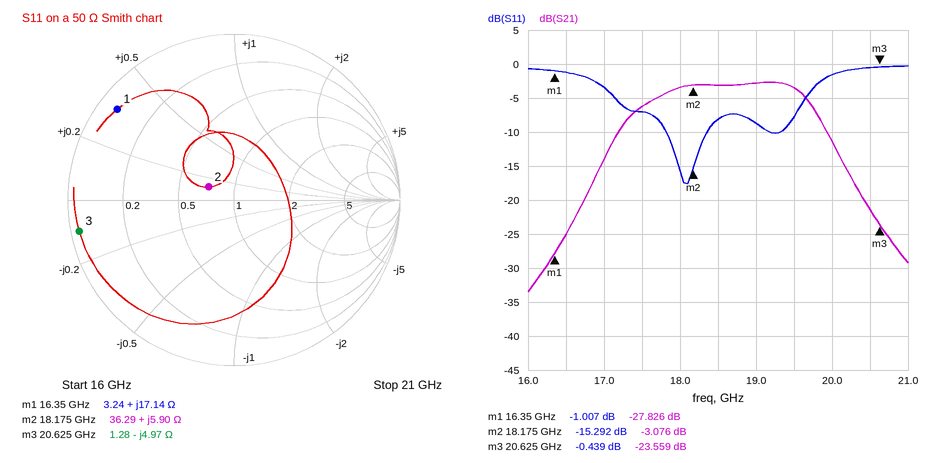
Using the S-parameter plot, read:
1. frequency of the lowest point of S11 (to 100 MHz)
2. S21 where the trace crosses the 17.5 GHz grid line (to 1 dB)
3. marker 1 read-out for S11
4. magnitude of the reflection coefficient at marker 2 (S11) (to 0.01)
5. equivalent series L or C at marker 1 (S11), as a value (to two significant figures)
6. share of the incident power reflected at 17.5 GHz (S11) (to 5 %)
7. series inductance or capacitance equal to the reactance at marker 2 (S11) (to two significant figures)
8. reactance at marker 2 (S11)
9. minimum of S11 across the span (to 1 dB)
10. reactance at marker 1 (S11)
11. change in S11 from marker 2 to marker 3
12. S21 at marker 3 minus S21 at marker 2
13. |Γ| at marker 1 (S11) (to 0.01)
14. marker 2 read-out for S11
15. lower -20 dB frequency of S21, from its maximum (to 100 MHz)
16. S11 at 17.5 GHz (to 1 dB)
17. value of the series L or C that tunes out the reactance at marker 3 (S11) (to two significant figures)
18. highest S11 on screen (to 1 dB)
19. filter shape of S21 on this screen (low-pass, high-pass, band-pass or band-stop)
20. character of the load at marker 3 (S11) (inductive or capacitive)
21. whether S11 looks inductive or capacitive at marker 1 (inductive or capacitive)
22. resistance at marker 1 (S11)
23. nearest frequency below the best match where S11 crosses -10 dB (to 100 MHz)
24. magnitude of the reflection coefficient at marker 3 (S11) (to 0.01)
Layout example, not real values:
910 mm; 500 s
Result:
18.1 GHz; -6 dB; -1.007 dB; 0.17; 170 pH; 20 %; 52 pH; +5.90 Ω; -18 dB; +17.14 Ω; 14.853 dB; -20.483 dB; 0.89; -15.292 dB; 16.6 GHz; -7 dB; 38 pH; 0 dB; band-pass; capacitive; inductive; 3.24 Ω; 17.8 GHz; 0.95
